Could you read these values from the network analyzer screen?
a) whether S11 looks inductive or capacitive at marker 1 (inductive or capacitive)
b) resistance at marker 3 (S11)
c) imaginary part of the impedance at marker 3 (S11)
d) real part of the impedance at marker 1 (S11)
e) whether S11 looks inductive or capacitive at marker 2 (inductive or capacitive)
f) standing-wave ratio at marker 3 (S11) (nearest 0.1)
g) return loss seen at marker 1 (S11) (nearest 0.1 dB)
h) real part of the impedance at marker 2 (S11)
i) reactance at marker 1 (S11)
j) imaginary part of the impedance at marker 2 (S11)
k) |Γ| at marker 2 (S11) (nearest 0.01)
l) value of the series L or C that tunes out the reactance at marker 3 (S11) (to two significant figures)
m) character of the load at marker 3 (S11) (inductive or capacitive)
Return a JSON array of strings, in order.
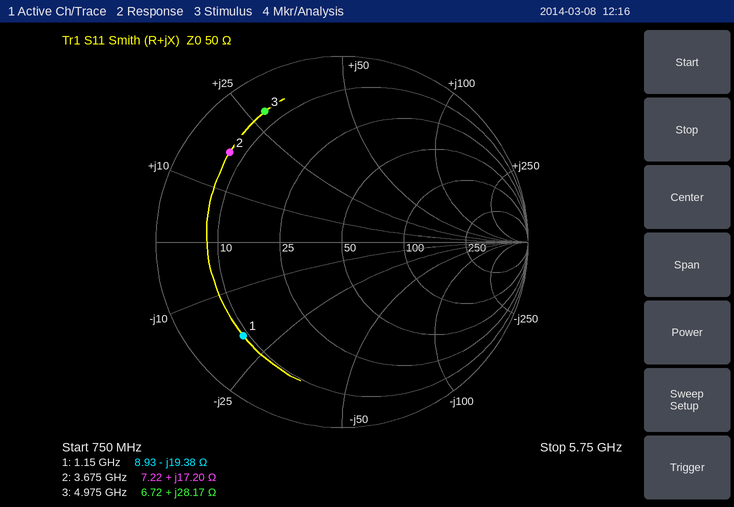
["capacitive", "6.72 Ω", "+28.17 Ω", "8.93 Ω", "inductive", "9.8", "2.7 dB", "7.22 Ω", "-19.38 Ω", "+17.20 Ω", "0.77", "1.1 pF", "inductive"]
